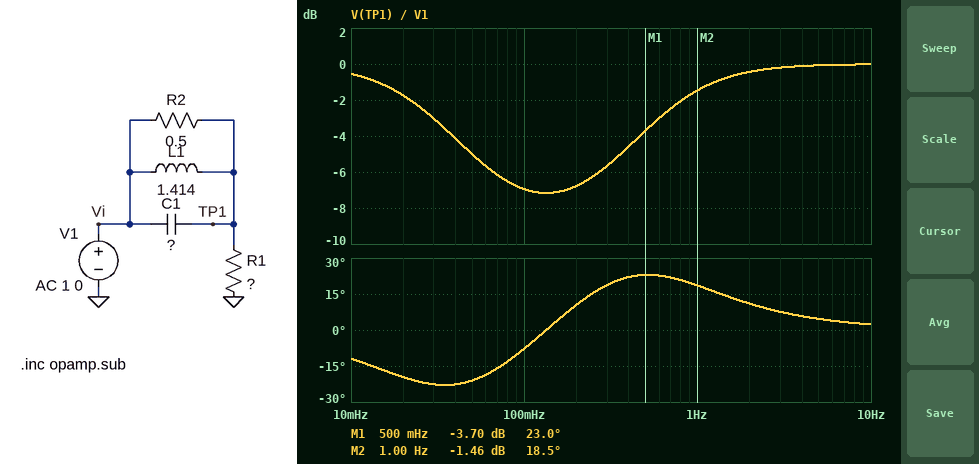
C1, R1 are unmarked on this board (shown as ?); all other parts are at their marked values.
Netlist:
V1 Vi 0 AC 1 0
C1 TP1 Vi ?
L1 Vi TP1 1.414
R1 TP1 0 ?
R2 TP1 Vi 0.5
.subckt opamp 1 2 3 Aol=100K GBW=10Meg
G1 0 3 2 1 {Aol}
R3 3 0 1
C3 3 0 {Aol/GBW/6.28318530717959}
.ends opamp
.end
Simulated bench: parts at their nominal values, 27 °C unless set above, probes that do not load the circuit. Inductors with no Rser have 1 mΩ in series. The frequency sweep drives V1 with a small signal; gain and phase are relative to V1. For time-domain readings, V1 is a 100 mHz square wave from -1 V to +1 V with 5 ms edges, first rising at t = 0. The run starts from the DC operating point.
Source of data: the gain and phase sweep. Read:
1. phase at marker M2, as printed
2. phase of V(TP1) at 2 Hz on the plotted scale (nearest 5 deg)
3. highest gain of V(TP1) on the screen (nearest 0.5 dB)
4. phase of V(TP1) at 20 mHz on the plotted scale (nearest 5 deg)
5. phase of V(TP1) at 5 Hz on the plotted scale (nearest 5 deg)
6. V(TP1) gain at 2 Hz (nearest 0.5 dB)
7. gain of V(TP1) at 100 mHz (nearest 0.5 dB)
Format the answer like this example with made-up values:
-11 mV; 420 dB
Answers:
18.5 deg; 10 deg; 0 dB; -20 deg; 5 deg; -0.5 dB; -7.0 dB
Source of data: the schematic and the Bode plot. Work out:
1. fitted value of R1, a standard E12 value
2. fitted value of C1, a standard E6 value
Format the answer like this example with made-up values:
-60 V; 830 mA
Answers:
0.39 Ω; 1 F
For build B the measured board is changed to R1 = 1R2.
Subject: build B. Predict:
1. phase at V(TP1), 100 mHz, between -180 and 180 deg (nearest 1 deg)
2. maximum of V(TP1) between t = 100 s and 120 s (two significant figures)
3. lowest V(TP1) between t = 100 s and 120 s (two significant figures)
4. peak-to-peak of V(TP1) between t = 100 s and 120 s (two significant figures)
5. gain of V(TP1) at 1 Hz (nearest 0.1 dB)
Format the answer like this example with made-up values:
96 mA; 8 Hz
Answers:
-4 deg; 1.1 V; -1.1 V; 2.3 V; -0.4 dB
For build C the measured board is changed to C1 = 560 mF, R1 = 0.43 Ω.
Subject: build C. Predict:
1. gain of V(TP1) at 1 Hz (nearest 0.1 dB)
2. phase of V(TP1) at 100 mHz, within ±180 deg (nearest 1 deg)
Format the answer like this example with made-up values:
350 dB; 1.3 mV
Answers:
-2.9 dB; -11 deg
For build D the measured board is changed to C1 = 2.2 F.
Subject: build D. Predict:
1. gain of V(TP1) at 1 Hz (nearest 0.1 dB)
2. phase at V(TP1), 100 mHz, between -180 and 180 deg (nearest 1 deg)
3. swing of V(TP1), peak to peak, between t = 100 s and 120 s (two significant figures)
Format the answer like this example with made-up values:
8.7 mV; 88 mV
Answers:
-0.4 dB; 4 deg; 2.8 V
